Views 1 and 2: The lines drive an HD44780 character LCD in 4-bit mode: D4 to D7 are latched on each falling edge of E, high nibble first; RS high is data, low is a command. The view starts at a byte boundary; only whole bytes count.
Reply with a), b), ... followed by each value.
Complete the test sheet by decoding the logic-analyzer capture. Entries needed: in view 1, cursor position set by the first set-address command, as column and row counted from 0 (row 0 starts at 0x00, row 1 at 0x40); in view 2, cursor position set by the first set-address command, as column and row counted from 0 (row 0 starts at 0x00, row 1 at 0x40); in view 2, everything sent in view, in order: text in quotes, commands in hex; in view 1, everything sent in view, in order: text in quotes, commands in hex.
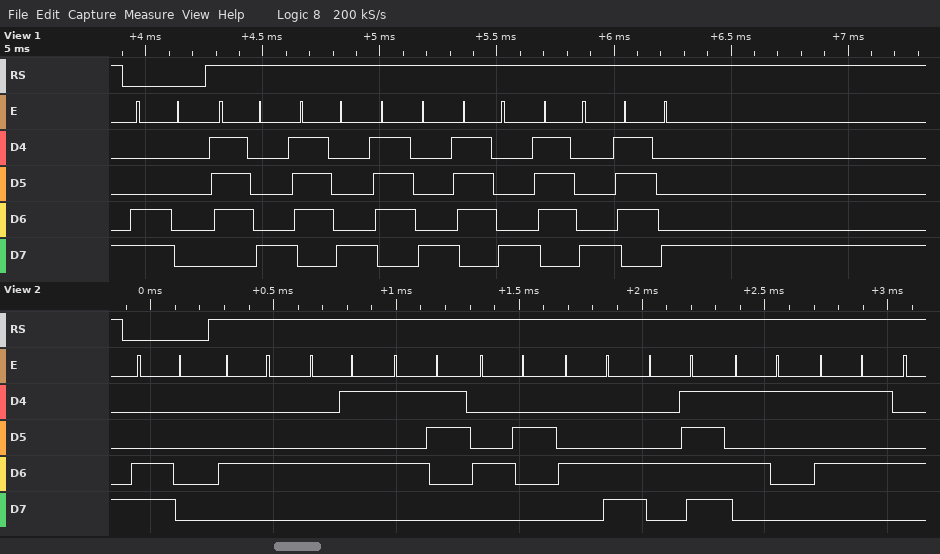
a) column 0, row 1
b) column 0, row 1
c) 0xC0 "DESBLOQU"
d) 0xC0 "xxxxxx"
